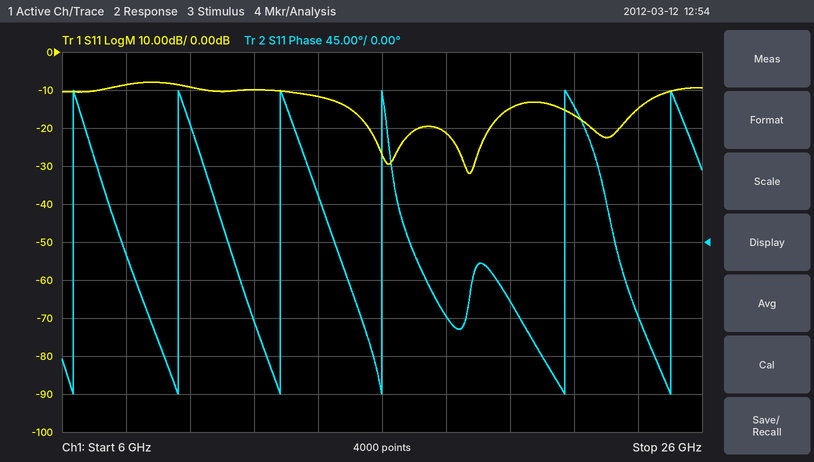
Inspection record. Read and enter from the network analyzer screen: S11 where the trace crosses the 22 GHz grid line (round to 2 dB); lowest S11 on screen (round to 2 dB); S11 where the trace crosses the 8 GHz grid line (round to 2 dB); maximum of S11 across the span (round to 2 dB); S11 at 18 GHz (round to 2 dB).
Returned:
-16 dB
-32 dB
-8 dB
-8 dB
-22 dB
